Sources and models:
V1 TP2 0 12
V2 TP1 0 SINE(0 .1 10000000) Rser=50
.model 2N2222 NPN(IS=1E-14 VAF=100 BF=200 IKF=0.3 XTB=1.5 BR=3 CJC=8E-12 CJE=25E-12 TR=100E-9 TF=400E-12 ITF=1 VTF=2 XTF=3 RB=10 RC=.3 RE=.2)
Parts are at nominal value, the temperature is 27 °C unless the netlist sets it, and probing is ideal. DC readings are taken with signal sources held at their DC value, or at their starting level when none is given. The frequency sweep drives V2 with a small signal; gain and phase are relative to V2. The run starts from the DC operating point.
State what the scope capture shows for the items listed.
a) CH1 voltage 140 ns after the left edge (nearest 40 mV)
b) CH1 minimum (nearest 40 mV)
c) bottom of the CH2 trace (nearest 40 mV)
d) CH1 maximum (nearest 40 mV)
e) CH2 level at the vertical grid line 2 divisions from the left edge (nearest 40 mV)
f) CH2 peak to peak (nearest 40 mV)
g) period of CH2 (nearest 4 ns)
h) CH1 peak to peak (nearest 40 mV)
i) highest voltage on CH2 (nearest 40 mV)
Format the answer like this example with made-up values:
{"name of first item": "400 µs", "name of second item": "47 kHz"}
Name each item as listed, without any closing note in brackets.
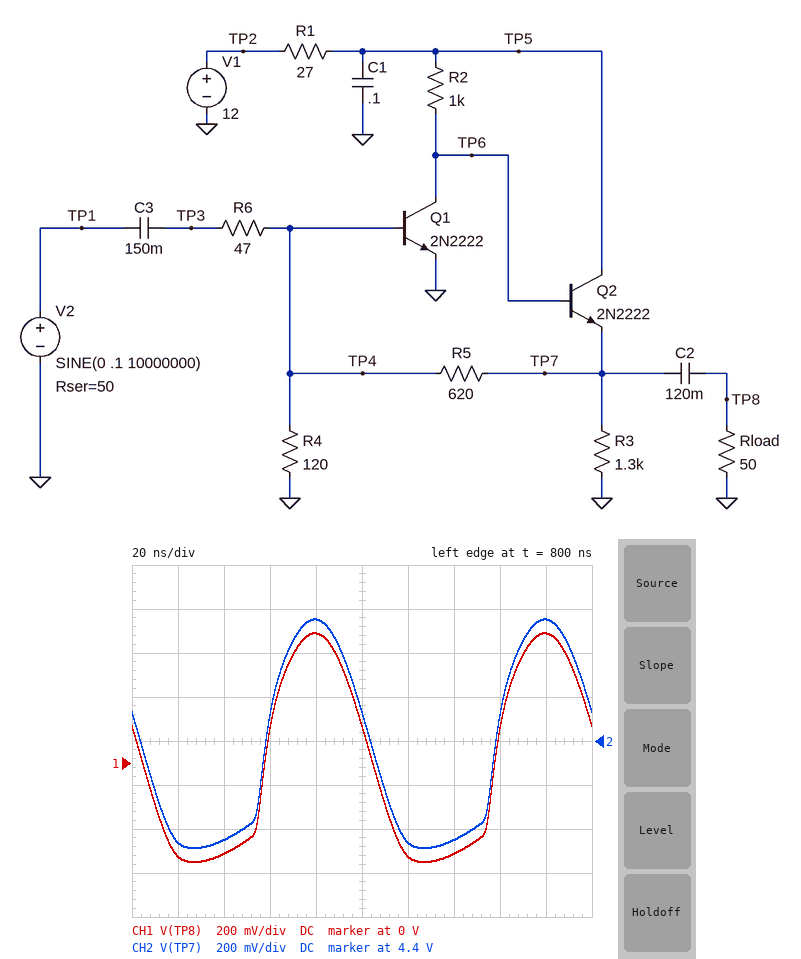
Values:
{"CH1 voltage 140 ns after the left edge": "-400 mV", "CH1 minimum": "-440 mV", "bottom of the CH2 trace": "3.92 V", "CH1 maximum": "600 mV", "CH2 level at the vertical grid line 2 divisions from the left edge": "3.96 V", "CH2 peak to peak": "1.04 V", "period of CH2": "100 ns", "CH1 peak to peak": "1.04 V", "highest voltage on CH2": "4.96 V"}
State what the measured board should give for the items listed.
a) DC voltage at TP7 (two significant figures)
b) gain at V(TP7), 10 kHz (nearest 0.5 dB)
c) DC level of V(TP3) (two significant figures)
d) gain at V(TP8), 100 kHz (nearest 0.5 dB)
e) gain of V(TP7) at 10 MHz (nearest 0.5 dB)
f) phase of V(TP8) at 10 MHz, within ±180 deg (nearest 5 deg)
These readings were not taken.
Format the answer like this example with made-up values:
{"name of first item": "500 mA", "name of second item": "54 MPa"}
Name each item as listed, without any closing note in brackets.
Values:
{"DC voltage at TP7": "4.4 V", "gain at V(TP7), 10 kHz": "15.5 dB", "DC level of V(TP3)": "700 mV", "gain at V(TP8), 100 kHz": "15.5 dB", "gain of V(TP7) at 10 MHz": "15.5 dB", "phase of V(TP8) at 10 MHz, within ±180 deg": "165 deg"}
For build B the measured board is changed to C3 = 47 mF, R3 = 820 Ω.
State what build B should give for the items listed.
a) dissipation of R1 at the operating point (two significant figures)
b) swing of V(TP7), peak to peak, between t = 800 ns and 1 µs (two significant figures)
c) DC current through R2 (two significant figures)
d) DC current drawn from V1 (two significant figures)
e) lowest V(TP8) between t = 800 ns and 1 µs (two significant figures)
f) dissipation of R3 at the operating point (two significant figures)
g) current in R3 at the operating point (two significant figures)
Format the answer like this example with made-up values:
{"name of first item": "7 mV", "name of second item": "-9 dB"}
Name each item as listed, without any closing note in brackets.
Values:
{"dissipation of R1 at the operating point": "8.4 mW", "swing of V(TP7), peak to peak, between t = 800 ns and 1 µs": "1.1 V", "DC current through R2": "6.4 mA", "DC current drawn from V1": "18 mA", "lowest V(TP8) between t = 800 ns and 1 µs": "-510 mV", "dissipation of R3 at the operating point": "23 mW", "current in R3 at the operating point": "5.3 mA"}
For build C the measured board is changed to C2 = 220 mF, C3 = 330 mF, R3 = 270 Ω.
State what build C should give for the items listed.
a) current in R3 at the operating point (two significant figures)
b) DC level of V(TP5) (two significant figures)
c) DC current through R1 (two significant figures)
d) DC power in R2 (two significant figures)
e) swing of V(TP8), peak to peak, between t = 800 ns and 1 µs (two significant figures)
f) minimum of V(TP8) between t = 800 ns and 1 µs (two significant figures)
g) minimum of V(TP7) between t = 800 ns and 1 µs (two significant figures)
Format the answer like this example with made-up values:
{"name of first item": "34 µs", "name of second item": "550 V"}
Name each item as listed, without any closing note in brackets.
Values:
{"current in R3 at the operating point": "16 mA", "DC level of V(TP5)": "11 V", "DC current through R1": "28 mA", "DC power in R2": "38 mW", "swing of V(TP8), peak to peak, between t = 800 ns and 1 µs": "1.2 V", "minimum of V(TP8) between t = 800 ns and 1 µs": "-590 mV", "minimum of V(TP7) between t = 800 ns and 1 µs": "3.8 V"}
